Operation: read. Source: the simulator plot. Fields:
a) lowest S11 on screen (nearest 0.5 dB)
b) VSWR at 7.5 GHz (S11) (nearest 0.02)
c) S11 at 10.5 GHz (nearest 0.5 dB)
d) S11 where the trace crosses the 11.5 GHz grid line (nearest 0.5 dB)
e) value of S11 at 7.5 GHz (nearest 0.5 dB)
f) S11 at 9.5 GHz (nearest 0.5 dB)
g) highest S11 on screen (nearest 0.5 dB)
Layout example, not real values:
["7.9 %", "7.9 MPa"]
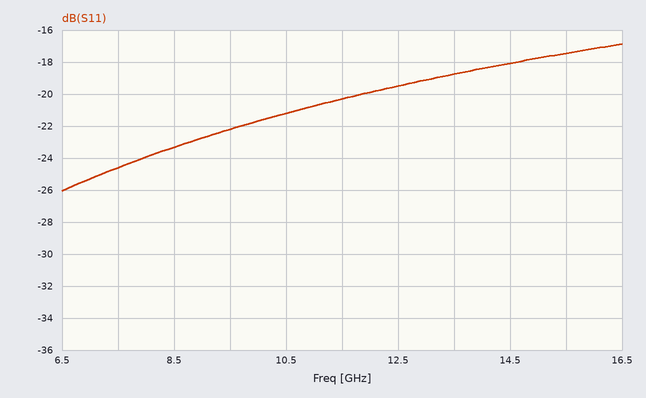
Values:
["-26.0 dB", "1.12", "-21.0 dB", "-20.5 dB", "-24.5 dB", "-22.0 dB", "-17.0 dB"]
